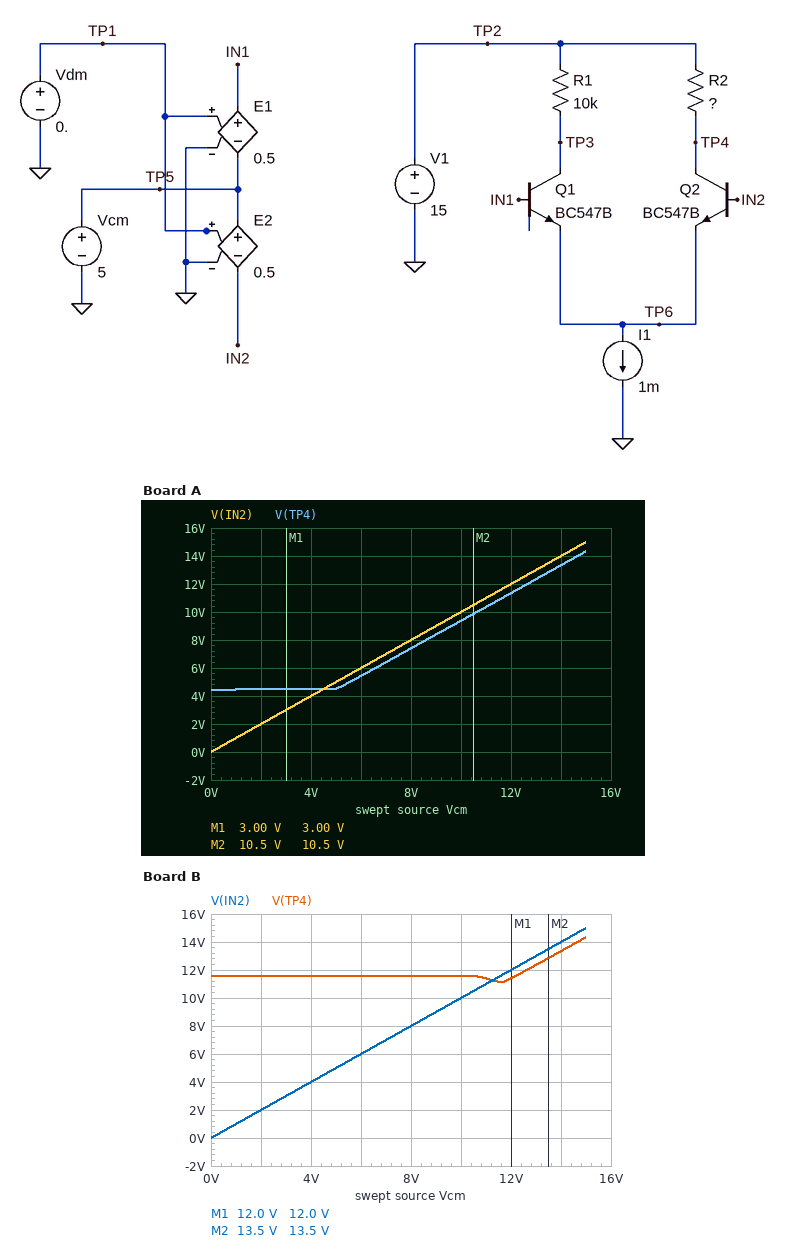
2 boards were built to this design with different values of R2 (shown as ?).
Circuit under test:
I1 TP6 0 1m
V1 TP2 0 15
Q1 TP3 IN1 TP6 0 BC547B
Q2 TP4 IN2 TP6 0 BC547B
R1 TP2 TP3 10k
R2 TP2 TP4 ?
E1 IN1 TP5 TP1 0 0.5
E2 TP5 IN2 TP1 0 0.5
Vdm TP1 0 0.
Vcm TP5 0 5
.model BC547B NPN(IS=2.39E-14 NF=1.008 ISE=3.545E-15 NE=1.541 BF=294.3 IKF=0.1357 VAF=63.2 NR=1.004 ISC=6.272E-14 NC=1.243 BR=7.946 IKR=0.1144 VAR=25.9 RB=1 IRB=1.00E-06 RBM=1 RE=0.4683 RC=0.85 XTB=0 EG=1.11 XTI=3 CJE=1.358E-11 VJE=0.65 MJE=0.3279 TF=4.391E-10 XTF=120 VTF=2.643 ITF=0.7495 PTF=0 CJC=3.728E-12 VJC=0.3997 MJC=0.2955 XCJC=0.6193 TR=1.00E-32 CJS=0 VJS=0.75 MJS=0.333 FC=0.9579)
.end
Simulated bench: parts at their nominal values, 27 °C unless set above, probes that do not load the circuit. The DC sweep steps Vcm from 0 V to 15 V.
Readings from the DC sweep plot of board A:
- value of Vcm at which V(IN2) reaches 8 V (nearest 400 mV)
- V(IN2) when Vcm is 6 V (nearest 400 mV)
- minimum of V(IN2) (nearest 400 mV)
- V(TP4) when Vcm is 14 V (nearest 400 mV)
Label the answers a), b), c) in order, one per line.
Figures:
a) 8.0 V
b) 6.0 V
c) 0 V
d) 13.2 V
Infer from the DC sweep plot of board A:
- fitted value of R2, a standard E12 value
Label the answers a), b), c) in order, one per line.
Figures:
a) 22 kΩ
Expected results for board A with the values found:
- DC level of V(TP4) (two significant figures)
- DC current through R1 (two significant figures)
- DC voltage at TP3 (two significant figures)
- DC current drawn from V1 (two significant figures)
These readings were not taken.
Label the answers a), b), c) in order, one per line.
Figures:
a) 4.5 V
b) 520 µA
c) 9.8 V
d) 1.0 mA
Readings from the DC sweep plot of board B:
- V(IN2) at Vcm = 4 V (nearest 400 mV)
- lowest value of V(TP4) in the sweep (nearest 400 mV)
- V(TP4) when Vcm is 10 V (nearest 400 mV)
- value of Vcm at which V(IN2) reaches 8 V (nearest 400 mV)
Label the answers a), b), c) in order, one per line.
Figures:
a) 4.0 V
b) 11.2 V
c) 11.6 V
d) 8.0 V
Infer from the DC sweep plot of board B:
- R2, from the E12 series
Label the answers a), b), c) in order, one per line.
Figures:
a) 6.8 kΩ
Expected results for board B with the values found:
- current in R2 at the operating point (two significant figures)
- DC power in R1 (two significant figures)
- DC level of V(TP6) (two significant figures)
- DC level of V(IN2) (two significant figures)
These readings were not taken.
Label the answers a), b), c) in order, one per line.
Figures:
a) 500 µA
b) 2.4 mW
c) 4.4 V
d) 5.0 V
